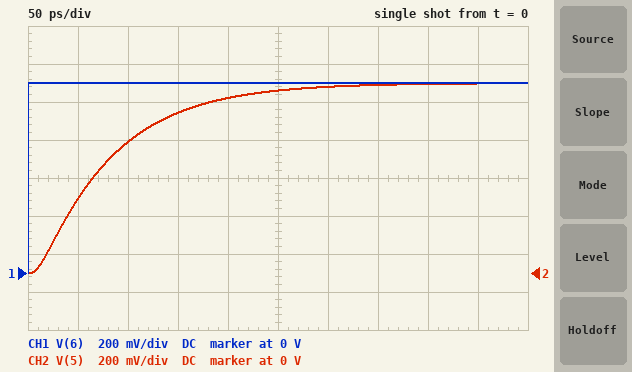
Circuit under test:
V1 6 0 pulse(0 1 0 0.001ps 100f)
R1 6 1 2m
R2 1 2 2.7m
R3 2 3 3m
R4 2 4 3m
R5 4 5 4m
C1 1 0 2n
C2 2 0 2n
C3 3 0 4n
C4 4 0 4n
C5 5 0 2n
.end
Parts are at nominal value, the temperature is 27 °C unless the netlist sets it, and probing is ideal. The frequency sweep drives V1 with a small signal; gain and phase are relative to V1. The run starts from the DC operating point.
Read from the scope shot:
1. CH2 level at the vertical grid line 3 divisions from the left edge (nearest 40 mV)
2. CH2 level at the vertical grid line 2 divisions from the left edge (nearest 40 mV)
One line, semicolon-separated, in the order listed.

840 mV; 680 mV
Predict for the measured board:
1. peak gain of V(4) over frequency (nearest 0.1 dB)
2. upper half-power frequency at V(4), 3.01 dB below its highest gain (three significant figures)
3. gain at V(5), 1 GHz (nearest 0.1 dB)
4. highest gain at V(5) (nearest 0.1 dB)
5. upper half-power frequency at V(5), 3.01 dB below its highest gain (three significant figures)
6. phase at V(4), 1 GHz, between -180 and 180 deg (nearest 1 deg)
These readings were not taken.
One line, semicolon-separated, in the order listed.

0 dB; 2.15 GHz; -0.9 dB; 0 dB; 2.12 GHz; -27 deg
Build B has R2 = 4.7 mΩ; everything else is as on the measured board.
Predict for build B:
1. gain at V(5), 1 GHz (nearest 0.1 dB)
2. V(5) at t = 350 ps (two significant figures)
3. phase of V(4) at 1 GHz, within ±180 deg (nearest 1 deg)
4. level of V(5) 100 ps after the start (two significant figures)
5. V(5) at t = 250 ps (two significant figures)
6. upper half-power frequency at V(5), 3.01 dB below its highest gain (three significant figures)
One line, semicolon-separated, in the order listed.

-1.4 dB; 970 mV; -33 deg; 590 mV; 910 mV; 1.62 GHz
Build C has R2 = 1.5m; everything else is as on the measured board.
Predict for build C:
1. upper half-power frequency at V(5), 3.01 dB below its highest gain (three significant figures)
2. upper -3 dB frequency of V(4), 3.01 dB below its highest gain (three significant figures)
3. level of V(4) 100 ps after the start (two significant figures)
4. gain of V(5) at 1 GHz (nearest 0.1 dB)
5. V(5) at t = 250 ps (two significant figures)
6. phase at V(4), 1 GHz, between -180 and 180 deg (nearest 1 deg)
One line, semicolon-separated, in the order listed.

2.59 GHz; 2.63 GHz; 800 mV; -0.6 dB; 980 mV; -22 deg
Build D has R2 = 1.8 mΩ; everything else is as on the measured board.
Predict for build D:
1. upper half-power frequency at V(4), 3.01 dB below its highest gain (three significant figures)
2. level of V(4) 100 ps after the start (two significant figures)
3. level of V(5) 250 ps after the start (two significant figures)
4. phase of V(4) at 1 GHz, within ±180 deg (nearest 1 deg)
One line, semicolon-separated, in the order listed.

2.49 GHz; 780 mV; 980 mV; -23 deg
